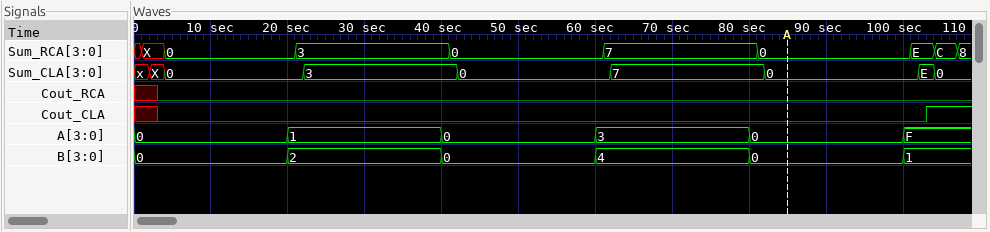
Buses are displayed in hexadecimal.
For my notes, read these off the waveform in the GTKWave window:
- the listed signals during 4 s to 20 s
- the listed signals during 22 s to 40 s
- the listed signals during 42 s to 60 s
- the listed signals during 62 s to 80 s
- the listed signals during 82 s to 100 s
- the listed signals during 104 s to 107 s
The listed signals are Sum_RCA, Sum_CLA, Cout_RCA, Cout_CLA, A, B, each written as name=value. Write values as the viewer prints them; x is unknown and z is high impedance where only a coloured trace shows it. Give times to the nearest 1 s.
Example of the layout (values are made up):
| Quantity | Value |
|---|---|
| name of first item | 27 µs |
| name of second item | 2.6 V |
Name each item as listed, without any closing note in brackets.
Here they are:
| Quantity | Value |
|---|---|
| the listed signals during 4 s to 20 s | Sum_RCA=0, Sum_CLA=0, Cout_RCA=0, Cout_CLA=0, A=0, B=0 |
| the listed signals during 22 s to 40 s | Sum_RCA=3, Sum_CLA=3, Cout_RCA=0, Cout_CLA=0, A=1, B=2 |
| the listed signals during 42 s to 60 s | Sum_RCA=0, Sum_CLA=0, Cout_RCA=0, Cout_CLA=0, A=0, B=0 |
| the listed signals during 62 s to 80 s | Sum_RCA=7, Sum_CLA=7, Cout_RCA=0, Cout_CLA=0, A=3, B=4 |
| the listed signals during 82 s to 100 s | Sum_RCA=0, Sum_CLA=0, Cout_RCA=0, Cout_CLA=0, A=0, B=0 |
| the listed signals during 104 s to 107 s | Sum_RCA=C, Sum_CLA=0, Cout_RCA=0, Cout_CLA=1, A=F, B=1 |
